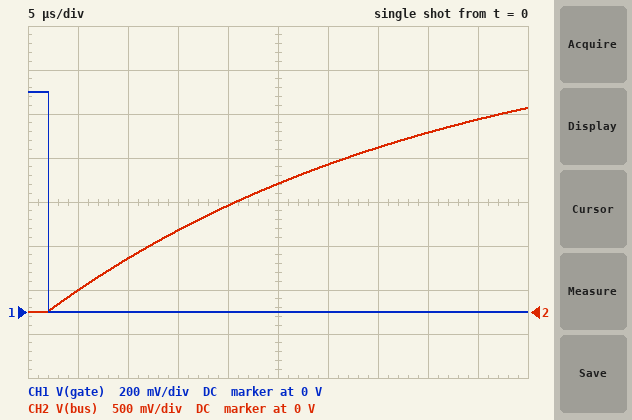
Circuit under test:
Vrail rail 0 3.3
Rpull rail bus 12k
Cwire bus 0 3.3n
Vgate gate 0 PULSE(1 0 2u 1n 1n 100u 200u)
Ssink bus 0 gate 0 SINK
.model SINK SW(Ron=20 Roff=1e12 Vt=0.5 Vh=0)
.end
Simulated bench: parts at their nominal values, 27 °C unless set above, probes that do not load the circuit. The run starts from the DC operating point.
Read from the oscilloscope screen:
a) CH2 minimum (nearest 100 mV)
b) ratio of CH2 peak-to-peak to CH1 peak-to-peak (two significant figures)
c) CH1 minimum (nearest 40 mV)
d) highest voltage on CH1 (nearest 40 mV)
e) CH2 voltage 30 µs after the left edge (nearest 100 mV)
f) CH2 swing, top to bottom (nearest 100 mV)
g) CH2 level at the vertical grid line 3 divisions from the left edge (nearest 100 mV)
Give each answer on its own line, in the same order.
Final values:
0 V
2.3
0 V
1.00 V
1.7 V
2.3 V
900 mV
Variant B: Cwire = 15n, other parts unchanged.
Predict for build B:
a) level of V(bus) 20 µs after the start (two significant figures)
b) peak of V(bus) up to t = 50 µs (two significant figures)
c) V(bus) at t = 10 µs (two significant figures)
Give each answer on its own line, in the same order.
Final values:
320 mV
780 mV
150 mV
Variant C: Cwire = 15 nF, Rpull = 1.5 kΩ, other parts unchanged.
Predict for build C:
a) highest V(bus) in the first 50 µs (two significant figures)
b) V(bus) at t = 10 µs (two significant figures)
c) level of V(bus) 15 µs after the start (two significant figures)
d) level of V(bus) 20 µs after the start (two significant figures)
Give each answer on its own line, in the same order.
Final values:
2.9 V
1.0 V
1.5 V
1.8 V
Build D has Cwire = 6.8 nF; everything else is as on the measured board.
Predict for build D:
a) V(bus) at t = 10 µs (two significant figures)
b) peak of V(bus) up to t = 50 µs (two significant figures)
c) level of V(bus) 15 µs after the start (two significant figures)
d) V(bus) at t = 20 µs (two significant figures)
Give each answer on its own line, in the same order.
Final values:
310 mV
1.5 V
490 mV
660 mV
